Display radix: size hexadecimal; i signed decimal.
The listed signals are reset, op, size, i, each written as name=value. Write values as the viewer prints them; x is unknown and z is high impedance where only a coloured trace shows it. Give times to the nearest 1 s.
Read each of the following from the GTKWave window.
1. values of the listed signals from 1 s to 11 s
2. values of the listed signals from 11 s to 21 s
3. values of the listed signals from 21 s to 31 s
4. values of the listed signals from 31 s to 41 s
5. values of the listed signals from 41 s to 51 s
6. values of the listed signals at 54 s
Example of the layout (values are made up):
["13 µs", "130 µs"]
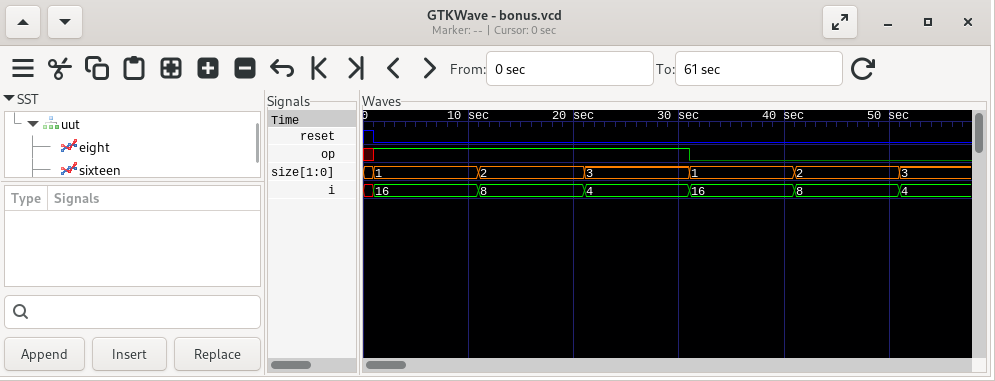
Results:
["reset=0, op=1, size=1, i=16", "reset=0, op=1, size=2, i=8", "reset=0, op=1, size=3, i=4", "reset=0, op=0, size=1, i=16", "reset=0, op=0, size=2, i=8", "reset=0, op=0, size=3, i=4"]
